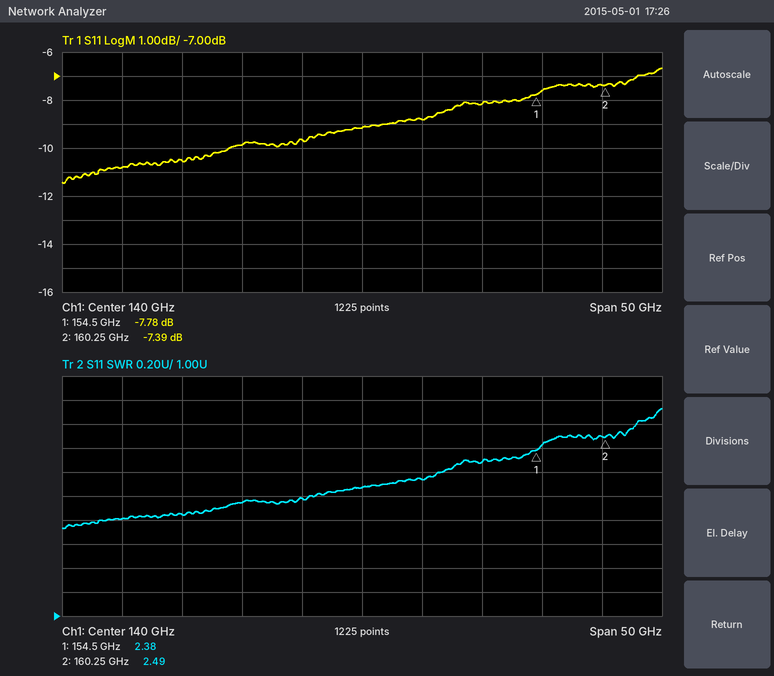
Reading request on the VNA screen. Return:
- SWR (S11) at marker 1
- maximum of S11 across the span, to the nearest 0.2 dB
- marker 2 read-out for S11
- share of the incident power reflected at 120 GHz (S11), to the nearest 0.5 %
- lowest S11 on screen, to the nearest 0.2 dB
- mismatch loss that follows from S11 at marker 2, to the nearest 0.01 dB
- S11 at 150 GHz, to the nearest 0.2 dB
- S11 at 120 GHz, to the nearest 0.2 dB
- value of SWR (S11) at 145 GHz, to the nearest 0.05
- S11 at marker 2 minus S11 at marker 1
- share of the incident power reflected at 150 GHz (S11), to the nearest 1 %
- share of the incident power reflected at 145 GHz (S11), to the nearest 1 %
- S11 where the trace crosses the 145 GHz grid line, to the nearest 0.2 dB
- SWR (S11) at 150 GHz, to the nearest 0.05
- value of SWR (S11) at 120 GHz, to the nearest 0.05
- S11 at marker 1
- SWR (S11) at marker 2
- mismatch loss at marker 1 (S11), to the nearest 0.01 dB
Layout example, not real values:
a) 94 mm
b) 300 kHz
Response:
a) 2.38
b) -6.6 dB
c) -7.39 dB
d) 8.5 %
e) -11.4 dB
f) 0.87 dB
g) -8.2 dB
h) -10.8 dB
i) 2.15
j) 0.39 dB
k) 15 %
l) 13 %
m) -8.8 dB
n) 2.30
o) 1.80
p) -7.78 dB
q) 2.49
r) 0.79 dB
